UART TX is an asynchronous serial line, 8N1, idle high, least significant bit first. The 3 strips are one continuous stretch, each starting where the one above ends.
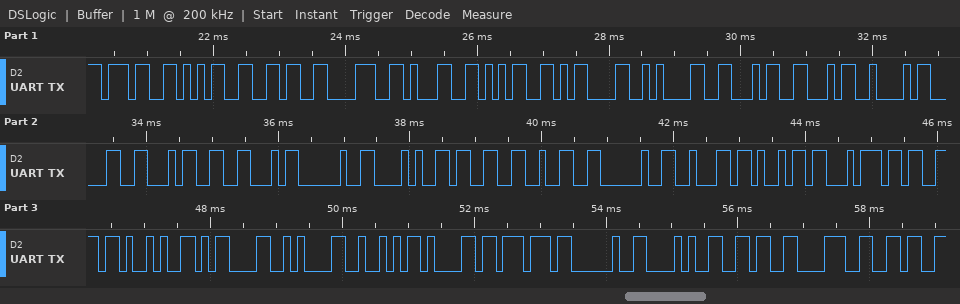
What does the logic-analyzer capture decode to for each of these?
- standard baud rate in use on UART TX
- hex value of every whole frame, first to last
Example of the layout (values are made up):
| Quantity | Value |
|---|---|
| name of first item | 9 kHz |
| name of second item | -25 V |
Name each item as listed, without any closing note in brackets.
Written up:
| Quantity | Value |
|---|---|
| standard baud rate in use on UART TX | 9600 baud |
| hex value of every whole frame, first to last | 37 35 36 38 31 35 0D 0A 46 46 42 30 34 46 20 28 33 32 20 62 69 74 73 29 0D 0A 52 61 77 20 28 36 38 36 |
